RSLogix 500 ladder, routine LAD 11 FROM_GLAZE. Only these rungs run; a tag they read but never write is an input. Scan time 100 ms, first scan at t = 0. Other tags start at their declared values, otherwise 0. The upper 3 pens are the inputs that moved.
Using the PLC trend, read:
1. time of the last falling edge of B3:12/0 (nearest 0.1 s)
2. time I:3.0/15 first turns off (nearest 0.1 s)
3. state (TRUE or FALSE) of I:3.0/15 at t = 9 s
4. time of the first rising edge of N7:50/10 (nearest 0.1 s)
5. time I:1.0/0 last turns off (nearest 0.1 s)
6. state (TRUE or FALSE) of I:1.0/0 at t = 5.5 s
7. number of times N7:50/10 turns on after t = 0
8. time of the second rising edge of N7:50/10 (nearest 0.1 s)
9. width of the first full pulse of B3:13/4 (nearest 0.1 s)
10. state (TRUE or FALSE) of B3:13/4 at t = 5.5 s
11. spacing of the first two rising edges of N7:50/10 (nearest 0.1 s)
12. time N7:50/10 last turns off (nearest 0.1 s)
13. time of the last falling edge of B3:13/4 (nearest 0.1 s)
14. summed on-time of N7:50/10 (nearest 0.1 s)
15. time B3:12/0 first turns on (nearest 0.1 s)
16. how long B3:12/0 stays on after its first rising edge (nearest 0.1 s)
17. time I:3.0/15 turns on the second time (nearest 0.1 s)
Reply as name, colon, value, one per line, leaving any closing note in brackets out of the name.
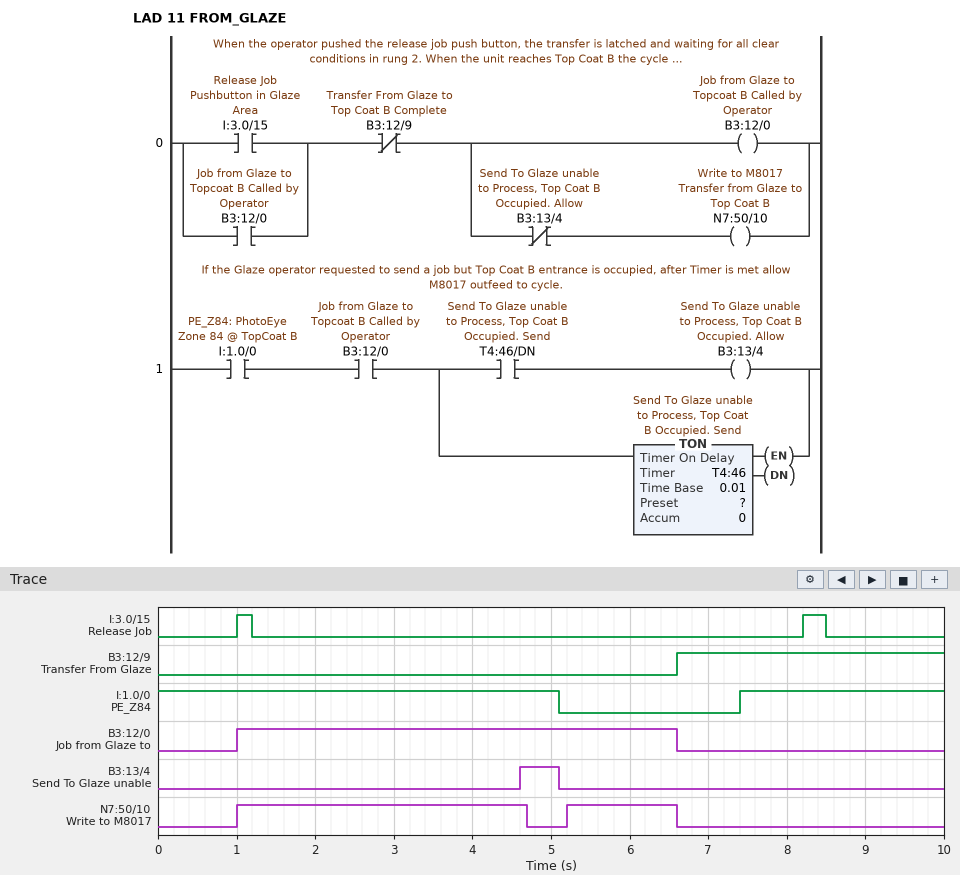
time of the last falling edge of B3:12/0: 6.6 s
time I:3.0/15 first turns off: 1.2 s
state (TRUE or FALSE) of I:3.0/15 at t = 9 s: FALSE
time of the first rising edge of N7:50/10: 1.0 s
time I:1.0/0 last turns off: 5.1 s
state (TRUE or FALSE) of I:1.0/0 at t = 5.5 s: FALSE
number of times N7:50/10 turns on after t = 0: 2
time of the second rising edge of N7:50/10: 5.2 s
width of the first full pulse of B3:13/4: 0.5 s
state (TRUE or FALSE) of B3:13/4 at t = 5.5 s: FALSE
spacing of the first two rising edges of N7:50/10: 4.2 s
time N7:50/10 last turns off: 6.6 s
time of the last falling edge of B3:13/4: 5.1 s
summed on-time of N7:50/10: 5.1 s
time B3:12/0 first turns on: 1.0 s
how long B3:12/0 stays on after its first rising edge: 5.6 s
time I:3.0/15 turns on the second time: 8.2 s
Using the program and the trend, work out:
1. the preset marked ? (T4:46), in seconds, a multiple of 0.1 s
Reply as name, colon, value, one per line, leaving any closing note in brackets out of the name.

the preset marked ? (T4:46), in seconds, a multiple of 0.1 s: 3.5 s
